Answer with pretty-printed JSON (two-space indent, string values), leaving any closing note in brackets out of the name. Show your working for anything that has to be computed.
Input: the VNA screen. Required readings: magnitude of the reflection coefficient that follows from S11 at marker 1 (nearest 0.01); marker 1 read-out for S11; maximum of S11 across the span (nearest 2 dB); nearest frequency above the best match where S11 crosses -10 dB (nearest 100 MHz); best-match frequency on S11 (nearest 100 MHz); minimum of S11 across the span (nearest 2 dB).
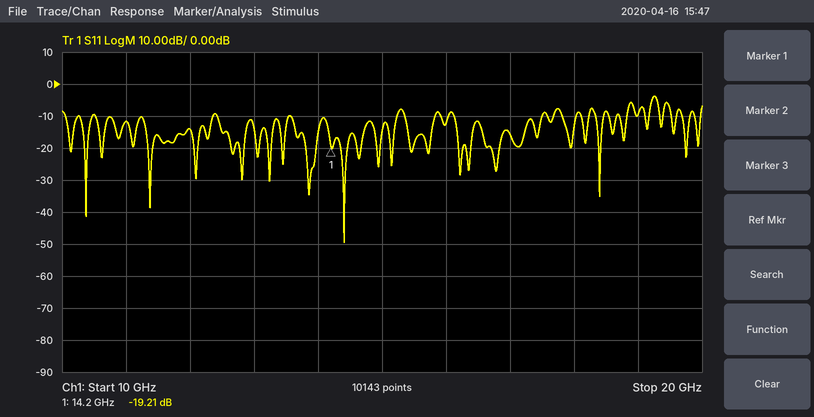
{
  "magnitude of the reflection coefficient that follows from S11 at marker 1": "10^(-19.21/20) ≈ 0.11",
  "marker 1 read-out for S11": "-19.21 dB",
  "maximum of S11 across the span": "-4 dB",
  "nearest frequency above the best match where S11 crosses -10 dB": "15.2 GHz",
  "best-match frequency on S11": "14.4 GHz",
  "minimum of S11 across the span": "-50 dB"
}
